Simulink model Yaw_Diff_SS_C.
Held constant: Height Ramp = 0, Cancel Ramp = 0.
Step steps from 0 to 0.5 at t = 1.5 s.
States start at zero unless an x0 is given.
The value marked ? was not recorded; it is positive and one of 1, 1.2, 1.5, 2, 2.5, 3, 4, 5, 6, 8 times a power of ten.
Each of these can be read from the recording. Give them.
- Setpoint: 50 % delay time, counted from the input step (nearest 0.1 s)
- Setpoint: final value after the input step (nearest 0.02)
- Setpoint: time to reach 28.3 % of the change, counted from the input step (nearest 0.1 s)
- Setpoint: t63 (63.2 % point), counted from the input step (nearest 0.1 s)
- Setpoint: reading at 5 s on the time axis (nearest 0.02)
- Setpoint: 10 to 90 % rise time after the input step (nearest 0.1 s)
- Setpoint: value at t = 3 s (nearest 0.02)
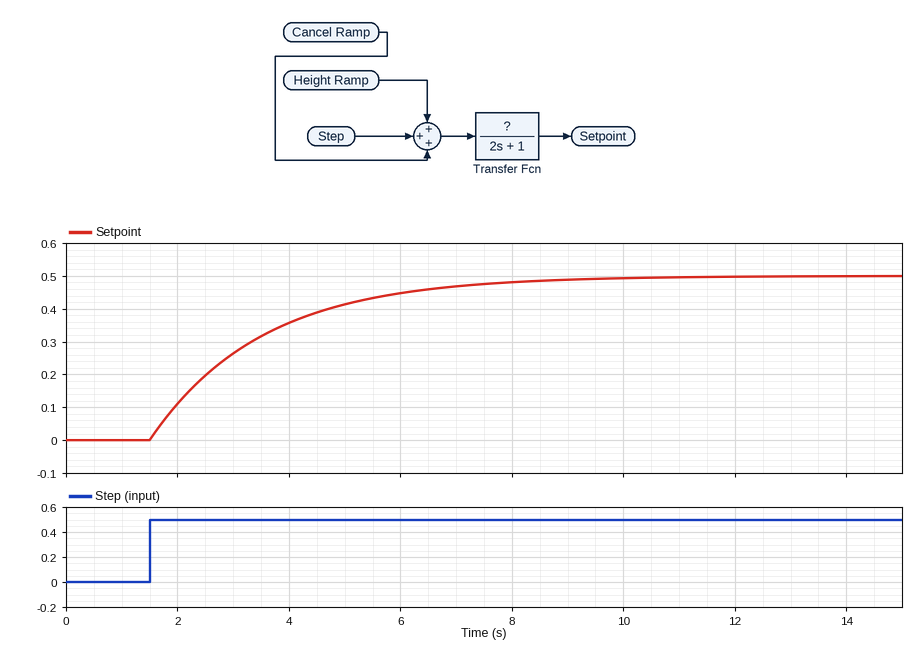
1.4 s
0.50
0.7 s
2.0 s
0.42
4.4 s
0.26
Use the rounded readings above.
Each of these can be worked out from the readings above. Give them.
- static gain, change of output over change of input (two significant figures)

1.0
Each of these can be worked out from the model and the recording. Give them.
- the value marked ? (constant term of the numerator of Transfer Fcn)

1
